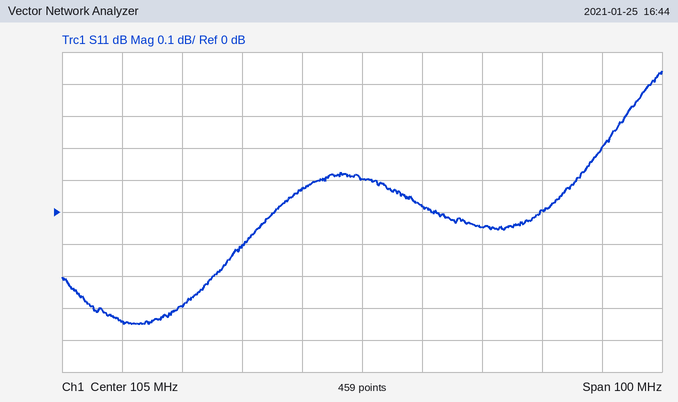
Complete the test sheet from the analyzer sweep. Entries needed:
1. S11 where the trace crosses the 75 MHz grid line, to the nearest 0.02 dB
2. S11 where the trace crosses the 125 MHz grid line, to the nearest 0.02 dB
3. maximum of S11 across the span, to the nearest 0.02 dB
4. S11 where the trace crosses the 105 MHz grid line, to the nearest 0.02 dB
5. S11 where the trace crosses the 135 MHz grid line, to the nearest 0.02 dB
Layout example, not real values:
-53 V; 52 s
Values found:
-0.30 dB; -0.04 dB; 0.44 dB; 0.10 dB; 0.00 dB
